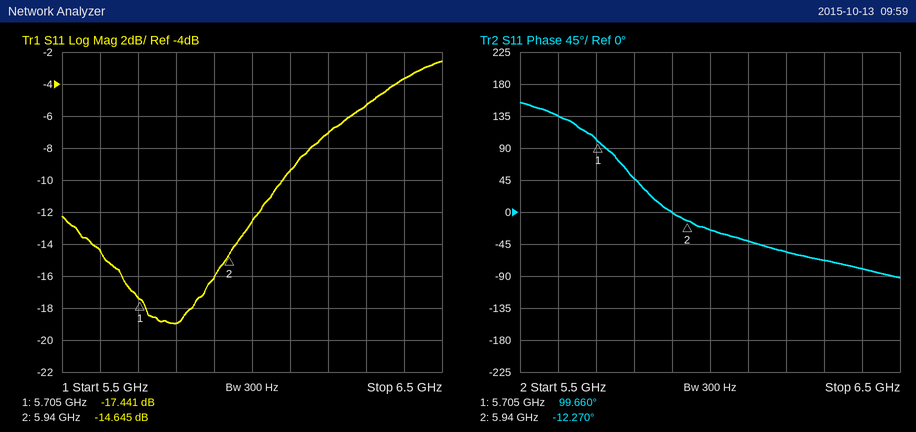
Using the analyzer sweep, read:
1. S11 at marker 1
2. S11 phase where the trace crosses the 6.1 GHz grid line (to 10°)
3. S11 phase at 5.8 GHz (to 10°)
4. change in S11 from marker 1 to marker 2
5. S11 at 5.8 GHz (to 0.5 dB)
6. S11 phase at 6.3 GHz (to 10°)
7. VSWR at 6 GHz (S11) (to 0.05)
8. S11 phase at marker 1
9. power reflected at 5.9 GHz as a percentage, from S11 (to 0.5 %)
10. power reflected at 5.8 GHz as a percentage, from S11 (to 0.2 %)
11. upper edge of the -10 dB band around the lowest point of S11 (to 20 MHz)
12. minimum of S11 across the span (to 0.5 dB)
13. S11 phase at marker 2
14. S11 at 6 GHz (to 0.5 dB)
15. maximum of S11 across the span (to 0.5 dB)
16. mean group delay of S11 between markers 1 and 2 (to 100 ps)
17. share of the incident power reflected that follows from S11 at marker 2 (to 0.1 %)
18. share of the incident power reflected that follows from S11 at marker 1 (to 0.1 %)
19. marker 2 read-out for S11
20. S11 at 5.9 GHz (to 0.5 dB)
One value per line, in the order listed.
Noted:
-17.441 dB
-40°
50°
2.796 dB
-19.0 dB
-70°
1.60
99.660°
2.5 %
1.2 %
6.08 GHz
-19.0 dB
-12.270°
-12.5 dB
-2.5 dB
1.3 ns
3.4 %
1.8 %
-14.645 dB
-16.0 dB
